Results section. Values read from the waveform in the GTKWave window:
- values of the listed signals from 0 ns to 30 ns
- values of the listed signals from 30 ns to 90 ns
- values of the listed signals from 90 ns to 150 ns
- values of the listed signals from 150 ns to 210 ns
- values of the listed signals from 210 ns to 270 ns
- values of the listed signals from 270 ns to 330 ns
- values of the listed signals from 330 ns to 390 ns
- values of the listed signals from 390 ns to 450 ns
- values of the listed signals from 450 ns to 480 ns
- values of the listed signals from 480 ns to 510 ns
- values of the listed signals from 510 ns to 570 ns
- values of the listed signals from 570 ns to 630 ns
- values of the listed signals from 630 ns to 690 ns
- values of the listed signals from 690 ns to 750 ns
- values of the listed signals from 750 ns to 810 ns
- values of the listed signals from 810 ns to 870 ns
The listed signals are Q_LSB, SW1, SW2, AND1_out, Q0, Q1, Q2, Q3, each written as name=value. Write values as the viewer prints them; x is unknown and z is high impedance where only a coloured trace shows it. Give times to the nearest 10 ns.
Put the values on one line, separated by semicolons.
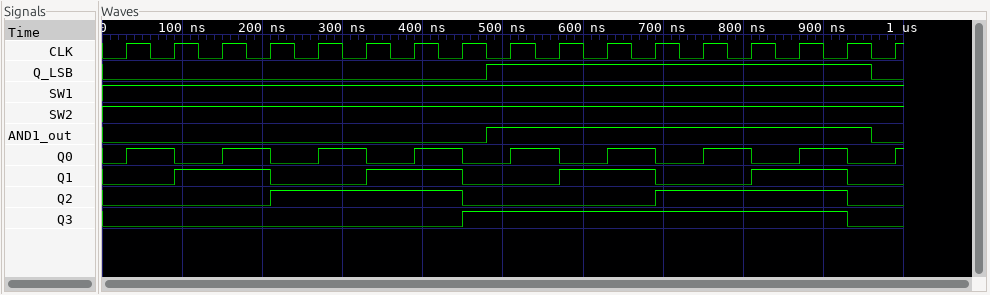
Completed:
Q_LSB=0, SW1=1, SW2=1, AND1_out=0, Q0=0, Q1=0, Q2=0, Q3=0; Q_LSB=0, SW1=1, SW2=1, AND1_out=0, Q0=1, Q1=0, Q2=0, Q3=0; Q_LSB=0, SW1=1, SW2=1, AND1_out=0, Q0=0, Q1=1, Q2=0, Q3=0; Q_LSB=0, SW1=1, SW2=1, AND1_out=0, Q0=1, Q1=1, Q2=0, Q3=0; Q_LSB=0, SW1=1, SW2=1, AND1_out=0, Q0=0, Q1=0, Q2=1, Q3=0; Q_LSB=0, SW1=1, SW2=1, AND1_out=0, Q0=1, Q1=0, Q2=1, Q3=0; Q_LSB=0, SW1=1, SW2=1, AND1_out=0, Q0=0, Q1=1, Q2=1, Q3=0; Q_LSB=0, SW1=1, SW2=1, AND1_out=0, Q0=1, Q1=1, Q2=1, Q3=0; Q_LSB=0, SW1=1, SW2=1, AND1_out=0, Q0=0, Q1=0, Q2=0, Q3=1; Q_LSB=1, SW1=1, SW2=1, AND1_out=1, Q0=0, Q1=0, Q2=0, Q3=1; Q_LSB=1, SW1=1, SW2=1, AND1_out=1, Q0=1, Q1=0, Q2=0, Q3=1; Q_LSB=1, SW1=1, SW2=1, AND1_out=1, Q0=0, Q1=1, Q2=0, Q3=1; Q_LSB=1, SW1=1, SW2=1, AND1_out=1, Q0=1, Q1=1, Q2=0, Q3=1; Q_LSB=1, SW1=1, SW2=1, AND1_out=1, Q0=0, Q1=0, Q2=1, Q3=1; Q_LSB=1, SW1=1, SW2=1, AND1_out=1, Q0=1, Q1=0, Q2=1, Q3=1; Q_LSB=1, SW1=1, SW2=1, AND1_out=1, Q0=0, Q1=1, Q2=1, Q3=1
